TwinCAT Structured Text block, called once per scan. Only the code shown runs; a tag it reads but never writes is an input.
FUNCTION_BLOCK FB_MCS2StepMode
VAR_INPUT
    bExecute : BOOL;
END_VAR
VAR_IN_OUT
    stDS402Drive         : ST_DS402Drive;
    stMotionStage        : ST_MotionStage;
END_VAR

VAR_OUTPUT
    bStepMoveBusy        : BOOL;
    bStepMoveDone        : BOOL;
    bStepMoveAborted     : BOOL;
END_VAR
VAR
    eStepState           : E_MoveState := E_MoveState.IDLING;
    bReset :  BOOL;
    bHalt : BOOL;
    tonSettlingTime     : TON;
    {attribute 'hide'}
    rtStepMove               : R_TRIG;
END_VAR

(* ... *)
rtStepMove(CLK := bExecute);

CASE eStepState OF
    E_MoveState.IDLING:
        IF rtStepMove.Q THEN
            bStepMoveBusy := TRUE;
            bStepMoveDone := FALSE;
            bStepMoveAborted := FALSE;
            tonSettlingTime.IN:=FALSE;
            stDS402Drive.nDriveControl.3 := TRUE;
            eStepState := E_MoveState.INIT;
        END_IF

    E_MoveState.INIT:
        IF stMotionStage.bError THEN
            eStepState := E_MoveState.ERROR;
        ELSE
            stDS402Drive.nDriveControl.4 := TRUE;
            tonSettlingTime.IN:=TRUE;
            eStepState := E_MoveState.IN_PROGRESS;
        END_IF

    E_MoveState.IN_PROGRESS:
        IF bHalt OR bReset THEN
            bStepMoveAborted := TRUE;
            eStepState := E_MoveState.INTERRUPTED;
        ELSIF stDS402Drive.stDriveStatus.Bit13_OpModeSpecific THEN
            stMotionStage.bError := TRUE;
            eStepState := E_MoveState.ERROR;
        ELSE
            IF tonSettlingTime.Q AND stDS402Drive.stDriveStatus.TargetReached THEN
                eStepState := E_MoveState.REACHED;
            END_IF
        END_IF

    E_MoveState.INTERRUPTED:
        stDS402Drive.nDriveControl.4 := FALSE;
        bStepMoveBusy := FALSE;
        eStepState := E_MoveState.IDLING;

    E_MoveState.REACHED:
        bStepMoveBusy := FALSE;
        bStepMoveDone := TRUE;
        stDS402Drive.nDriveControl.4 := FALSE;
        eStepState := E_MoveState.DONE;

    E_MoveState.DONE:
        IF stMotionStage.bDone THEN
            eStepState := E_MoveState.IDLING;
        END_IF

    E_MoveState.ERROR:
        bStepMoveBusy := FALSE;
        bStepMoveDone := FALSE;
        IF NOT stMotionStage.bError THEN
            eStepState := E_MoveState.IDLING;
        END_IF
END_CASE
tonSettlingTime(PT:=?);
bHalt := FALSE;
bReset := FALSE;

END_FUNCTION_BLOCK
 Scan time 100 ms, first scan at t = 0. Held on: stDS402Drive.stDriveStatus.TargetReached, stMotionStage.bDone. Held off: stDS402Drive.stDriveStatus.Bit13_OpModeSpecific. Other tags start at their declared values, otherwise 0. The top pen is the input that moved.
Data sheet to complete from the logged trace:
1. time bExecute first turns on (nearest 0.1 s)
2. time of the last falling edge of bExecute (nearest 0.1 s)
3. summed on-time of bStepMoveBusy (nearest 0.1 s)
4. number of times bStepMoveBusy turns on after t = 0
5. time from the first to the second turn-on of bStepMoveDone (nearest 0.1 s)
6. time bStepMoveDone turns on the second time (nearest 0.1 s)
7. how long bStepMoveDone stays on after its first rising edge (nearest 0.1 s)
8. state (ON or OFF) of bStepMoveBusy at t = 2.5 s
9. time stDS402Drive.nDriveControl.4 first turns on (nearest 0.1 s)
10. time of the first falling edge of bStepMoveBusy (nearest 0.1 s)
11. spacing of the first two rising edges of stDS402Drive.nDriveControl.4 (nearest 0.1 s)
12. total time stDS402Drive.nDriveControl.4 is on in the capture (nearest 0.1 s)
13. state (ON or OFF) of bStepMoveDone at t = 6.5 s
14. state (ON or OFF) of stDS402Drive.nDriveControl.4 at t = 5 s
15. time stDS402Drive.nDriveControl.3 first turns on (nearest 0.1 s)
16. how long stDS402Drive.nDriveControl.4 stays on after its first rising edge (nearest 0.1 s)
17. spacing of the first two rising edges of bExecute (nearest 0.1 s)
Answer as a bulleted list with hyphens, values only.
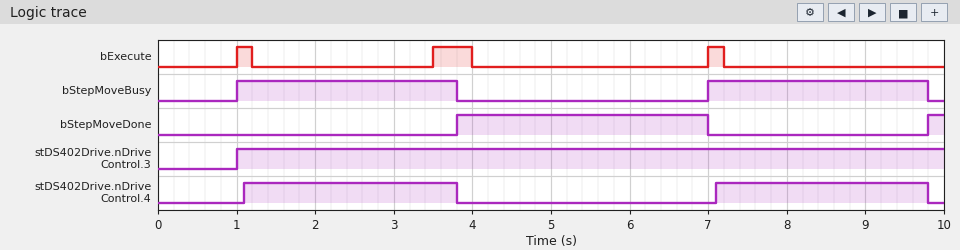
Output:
- 1.0 s
- 7.2 s
- 5.6 s
- 2
- 6.0 s
- 9.8 s
- 3.2 s
- ON
- 1.1 s
- 3.8 s
- 6.0 s
- 5.4 s
- ON
- OFF
- 1.0 s
- 2.7 s
- 2.5 s
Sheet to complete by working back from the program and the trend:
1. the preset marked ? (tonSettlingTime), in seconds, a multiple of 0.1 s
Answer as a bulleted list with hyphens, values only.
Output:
- 2.5 s
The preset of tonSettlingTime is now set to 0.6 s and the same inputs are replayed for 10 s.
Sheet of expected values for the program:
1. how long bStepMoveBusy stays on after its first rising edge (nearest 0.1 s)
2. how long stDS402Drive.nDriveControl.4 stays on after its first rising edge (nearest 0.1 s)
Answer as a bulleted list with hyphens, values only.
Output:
- 0.9 s
- 0.8 s
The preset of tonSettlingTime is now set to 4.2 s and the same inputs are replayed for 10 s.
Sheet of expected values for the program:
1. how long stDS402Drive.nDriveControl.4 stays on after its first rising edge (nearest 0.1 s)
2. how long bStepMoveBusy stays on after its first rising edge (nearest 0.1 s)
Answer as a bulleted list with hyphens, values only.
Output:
- 4.4 s
- 4.5 s
